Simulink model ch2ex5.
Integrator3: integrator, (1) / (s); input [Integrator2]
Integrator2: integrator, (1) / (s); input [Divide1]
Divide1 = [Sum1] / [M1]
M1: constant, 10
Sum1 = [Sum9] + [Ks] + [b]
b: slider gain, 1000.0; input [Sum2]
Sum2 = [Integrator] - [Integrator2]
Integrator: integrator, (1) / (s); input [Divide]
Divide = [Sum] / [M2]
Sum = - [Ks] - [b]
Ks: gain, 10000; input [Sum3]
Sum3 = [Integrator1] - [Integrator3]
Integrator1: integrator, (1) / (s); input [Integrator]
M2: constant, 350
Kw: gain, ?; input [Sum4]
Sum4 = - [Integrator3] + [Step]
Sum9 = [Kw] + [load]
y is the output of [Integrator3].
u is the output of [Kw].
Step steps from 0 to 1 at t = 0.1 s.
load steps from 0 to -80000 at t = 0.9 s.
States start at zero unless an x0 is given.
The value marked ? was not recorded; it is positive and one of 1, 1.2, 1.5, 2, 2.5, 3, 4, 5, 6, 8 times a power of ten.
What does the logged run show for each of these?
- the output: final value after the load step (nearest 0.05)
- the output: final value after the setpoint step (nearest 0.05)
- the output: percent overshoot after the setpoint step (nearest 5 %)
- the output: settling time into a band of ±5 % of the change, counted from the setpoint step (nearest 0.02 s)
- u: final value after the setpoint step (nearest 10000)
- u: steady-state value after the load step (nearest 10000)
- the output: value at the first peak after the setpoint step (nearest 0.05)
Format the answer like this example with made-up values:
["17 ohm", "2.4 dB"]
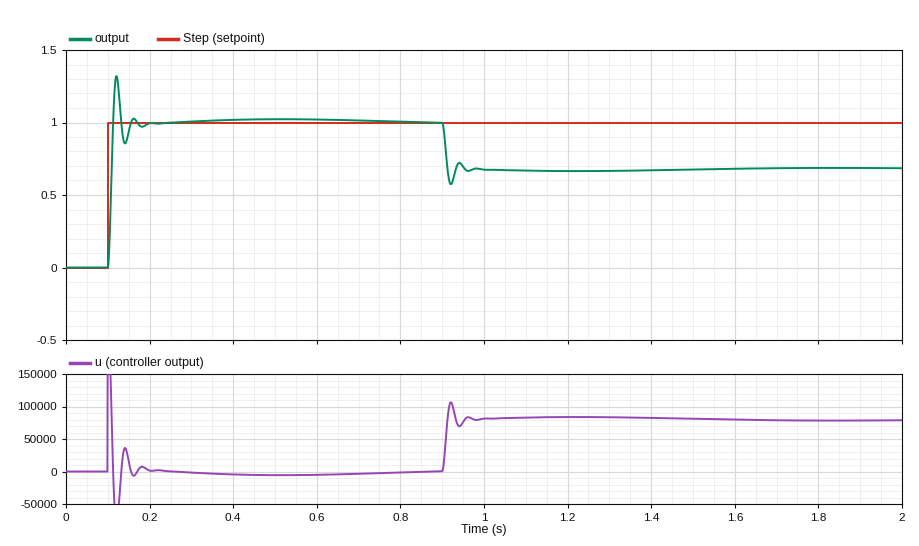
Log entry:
["0.70", "1.00", "30 %", "0.06 s", "0", "80000", "1.30"]
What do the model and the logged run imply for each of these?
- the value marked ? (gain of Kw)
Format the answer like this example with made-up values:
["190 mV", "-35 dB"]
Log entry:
["250000"]
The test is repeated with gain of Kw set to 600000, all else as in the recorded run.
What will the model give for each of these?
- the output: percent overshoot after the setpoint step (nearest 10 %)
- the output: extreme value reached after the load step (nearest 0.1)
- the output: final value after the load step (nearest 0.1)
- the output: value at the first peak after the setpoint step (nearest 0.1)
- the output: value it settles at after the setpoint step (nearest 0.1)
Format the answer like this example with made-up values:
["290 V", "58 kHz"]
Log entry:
["50 %", "0.8", "0.9", "1.5", "1.0"]
